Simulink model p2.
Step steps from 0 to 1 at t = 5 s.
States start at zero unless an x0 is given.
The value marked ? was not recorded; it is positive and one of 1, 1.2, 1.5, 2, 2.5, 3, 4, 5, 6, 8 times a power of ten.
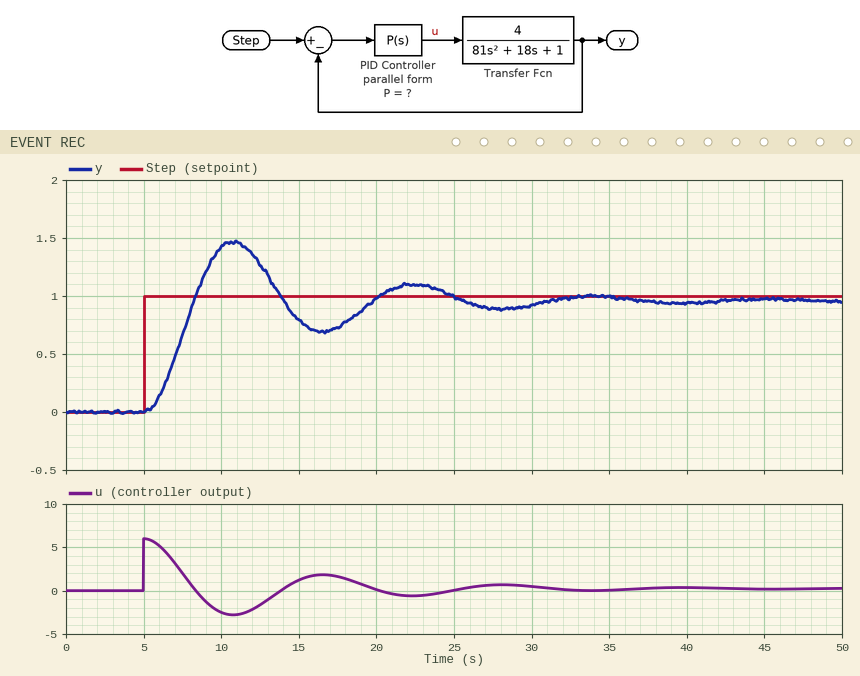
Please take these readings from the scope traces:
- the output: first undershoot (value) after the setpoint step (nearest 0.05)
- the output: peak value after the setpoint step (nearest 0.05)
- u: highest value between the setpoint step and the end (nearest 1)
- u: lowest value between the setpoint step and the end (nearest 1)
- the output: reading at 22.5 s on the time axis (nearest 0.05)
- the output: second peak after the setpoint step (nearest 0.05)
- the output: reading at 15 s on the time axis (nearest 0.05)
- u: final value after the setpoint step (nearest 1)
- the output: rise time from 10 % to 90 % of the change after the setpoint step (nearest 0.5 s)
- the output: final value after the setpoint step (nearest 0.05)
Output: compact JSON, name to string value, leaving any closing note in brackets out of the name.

{"the output: first undershoot (value) after the setpoint step": "0.70", "the output: peak value after the setpoint step": "1.45", "u: highest value between the setpoint step and the end": "6", "u: lowest value between the setpoint step and the end": "-3", "the output: reading at 22.5 s on the time axis": "1.10", "the output: second peak after the setpoint step": "1.10", "the output: reading at 15 s on the time axis": "0.80", "u: final value after the setpoint step": "0", "the output: rise time from 10 % to 90 % of the change after the setpoint step": "2.0 s", "the output: final value after the setpoint step": "0.95"}
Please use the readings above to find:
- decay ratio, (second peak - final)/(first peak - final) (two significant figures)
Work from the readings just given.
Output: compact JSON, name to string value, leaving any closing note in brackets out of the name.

{"decay ratio, (second peak - final)/(first peak - final)": "0.30"}
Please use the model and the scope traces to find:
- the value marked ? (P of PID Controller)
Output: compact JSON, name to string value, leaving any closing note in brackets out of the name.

{"the value marked ?": "6"}
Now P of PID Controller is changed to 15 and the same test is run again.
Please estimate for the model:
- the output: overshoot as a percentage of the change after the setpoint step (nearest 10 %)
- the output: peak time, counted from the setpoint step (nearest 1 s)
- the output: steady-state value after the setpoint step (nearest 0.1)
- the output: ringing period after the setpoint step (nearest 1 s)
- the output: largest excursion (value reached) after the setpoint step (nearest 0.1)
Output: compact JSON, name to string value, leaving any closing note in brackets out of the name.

{"the output: overshoot as a percentage of the change after the setpoint step": "70 %", "the output: peak time, counted from the setpoint step": "4 s", "the output: steady-state value after the setpoint step": "1.0", "the output: ringing period after the setpoint step": "7 s", "the output: largest excursion (value reached) after the setpoint step": "1.6"}
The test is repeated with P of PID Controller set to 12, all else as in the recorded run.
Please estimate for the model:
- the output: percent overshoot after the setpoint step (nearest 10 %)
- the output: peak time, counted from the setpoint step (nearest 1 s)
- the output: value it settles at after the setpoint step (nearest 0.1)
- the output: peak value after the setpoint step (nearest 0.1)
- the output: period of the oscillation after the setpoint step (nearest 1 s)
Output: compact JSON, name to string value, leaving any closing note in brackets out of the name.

{"the output: percent overshoot after the setpoint step": "60 %", "the output: peak time, counted from the setpoint step": "4 s", "the output: value it settles at after the setpoint step": "1.0", "the output: peak value after the setpoint step": "1.6", "the output: period of the oscillation after the setpoint step": "8 s"}
